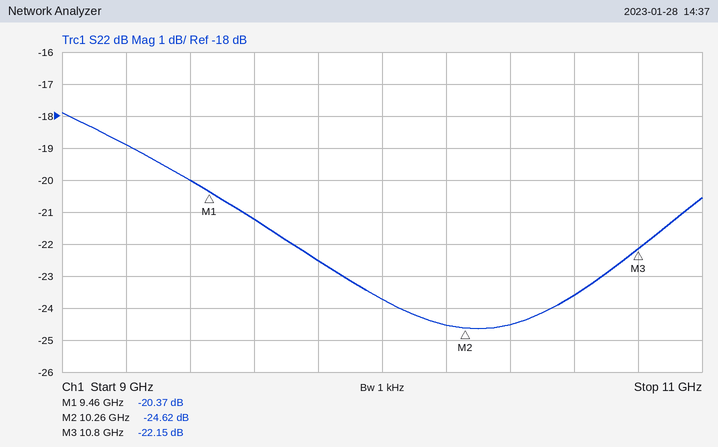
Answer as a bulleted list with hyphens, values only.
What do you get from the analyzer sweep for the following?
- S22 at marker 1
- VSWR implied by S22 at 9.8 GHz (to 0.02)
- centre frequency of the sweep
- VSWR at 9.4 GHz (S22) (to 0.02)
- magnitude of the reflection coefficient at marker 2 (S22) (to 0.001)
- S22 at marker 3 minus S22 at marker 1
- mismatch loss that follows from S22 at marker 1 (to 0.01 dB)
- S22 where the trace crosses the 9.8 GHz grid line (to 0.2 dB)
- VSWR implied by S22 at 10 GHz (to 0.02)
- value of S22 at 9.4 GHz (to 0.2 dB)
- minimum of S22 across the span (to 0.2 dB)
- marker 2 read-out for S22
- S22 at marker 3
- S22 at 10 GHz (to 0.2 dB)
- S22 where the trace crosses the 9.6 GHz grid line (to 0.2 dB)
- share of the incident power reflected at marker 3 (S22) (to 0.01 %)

- -20.37 dB
- 1.16
- 10 GHz
- 1.22
- 0.059
- -1.78 dB
- 0.04 dB
- -22.6 dB
- 1.14
- -20.0 dB
- -24.6 dB
- -24.62 dB
- -22.15 dB
- -23.8 dB
- -21.2 dB
- 0.61 %
